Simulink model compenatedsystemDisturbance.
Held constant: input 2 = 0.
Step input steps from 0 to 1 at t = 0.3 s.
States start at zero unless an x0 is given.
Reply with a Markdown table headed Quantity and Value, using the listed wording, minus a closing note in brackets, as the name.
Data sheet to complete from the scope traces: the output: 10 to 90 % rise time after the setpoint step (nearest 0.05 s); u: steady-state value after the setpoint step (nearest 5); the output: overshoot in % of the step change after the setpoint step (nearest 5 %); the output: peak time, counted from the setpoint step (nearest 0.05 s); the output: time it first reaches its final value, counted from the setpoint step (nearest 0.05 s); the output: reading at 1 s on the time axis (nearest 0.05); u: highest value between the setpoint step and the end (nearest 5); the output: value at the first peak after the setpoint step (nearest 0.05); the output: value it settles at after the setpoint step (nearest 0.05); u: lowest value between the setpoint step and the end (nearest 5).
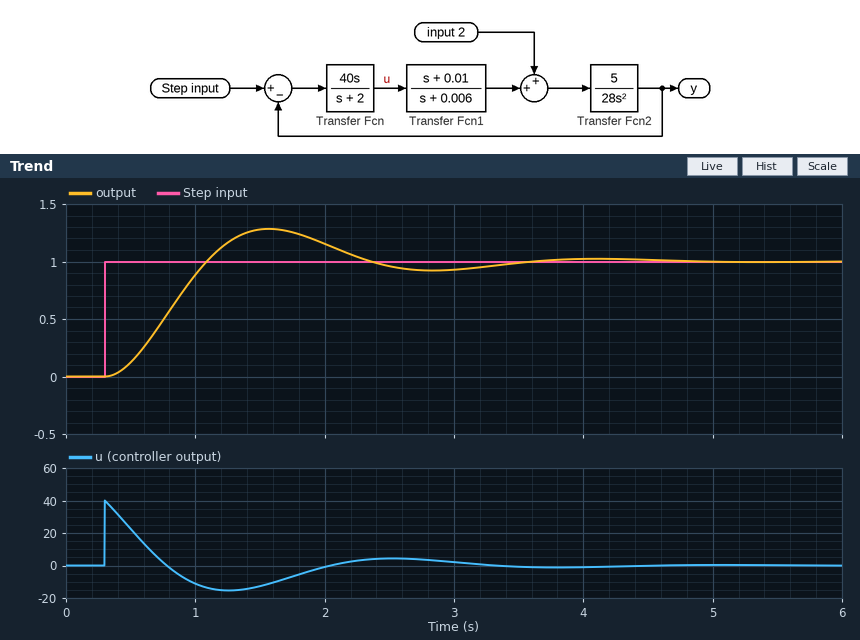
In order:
| Quantity | Value |
|---|---|
| the output: 10 to 90 % rise time after the setpoint step | 0.55 s |
| u: steady-state value after the setpoint step | 0 |
| the output: overshoot in % of the step change after the setpoint step | 30 % |
| the output: peak time, counted from the setpoint step | 1.25 s |
| the output: time it first reaches its final value, counted from the setpoint step | 0.80 s |
| the output: reading at 1 s on the time axis | 0.90 |
| u: highest value between the setpoint step and the end | 40 |
| the output: value at the first peak after the setpoint step | 1.30 |
| the output: value it settles at after the setpoint step | 1.00 |
| u: lowest value between the setpoint step and the end | -15 |
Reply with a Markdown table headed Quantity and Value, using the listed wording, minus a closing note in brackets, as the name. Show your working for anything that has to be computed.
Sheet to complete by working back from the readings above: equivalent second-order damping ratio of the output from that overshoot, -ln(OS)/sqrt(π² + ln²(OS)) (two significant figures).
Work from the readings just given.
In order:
| Quantity | Value |
|---|---|
| equivalent second-order damping ratio of the output from that overshoot, -ln(OS)/sqrt(π² + ln²(OS)) | ln(0.3) = -1.204; 1.204 / sqrt(9.870 + 1.450) = 0.36 |
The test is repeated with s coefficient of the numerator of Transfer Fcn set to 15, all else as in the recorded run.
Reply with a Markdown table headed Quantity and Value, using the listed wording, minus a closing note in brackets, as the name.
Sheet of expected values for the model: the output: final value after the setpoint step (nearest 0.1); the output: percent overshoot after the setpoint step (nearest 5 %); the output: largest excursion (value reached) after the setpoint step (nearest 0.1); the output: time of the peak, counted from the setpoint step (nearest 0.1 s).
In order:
| Quantity | Value |
|---|---|
| the output: final value after the setpoint step | 1.0 |
| the output: percent overshoot after the setpoint step | 10 % |
| the output: largest excursion (value reached) after the setpoint step | 1.1 |
| the output: time of the peak, counted from the setpoint step | 2.4 s |
